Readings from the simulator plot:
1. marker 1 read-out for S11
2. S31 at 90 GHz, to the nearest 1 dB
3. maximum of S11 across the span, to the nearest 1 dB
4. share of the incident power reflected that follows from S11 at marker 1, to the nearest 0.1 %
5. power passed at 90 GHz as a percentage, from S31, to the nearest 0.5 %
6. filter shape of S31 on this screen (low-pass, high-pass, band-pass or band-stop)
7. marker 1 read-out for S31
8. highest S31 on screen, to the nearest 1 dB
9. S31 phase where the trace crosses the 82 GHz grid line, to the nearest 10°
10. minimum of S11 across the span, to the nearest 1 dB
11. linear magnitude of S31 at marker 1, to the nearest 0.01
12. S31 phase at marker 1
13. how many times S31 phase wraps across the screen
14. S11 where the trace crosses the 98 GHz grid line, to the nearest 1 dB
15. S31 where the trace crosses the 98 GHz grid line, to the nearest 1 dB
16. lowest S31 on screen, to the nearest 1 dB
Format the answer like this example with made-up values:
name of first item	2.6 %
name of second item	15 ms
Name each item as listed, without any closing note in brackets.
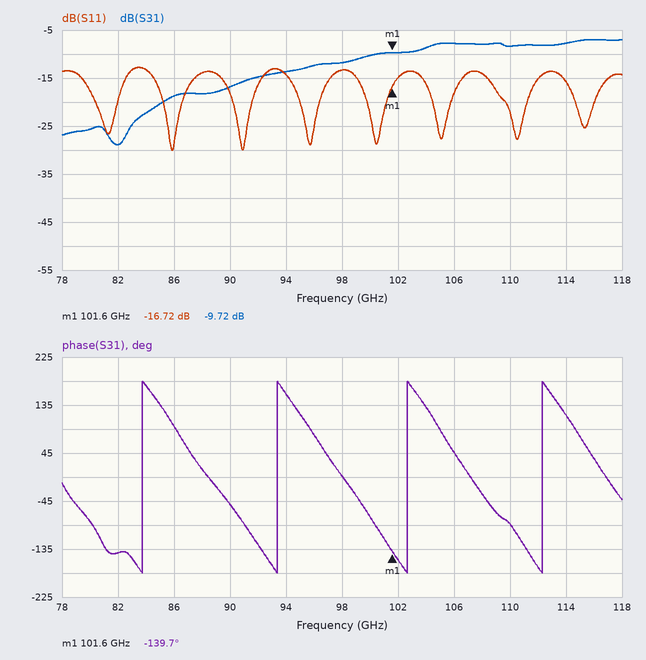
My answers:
marker 1 read-out for S11	-16.72 dB
S31 at 90 GHz, to the nearest 1 dB	-17 dB
maximum of S11 across the span, to the nearest 1 dB	-13 dB
share of the incident power reflected that follows from S11 at marker 1, to the nearest 0.1 %	2.1 %
power passed at 90 GHz as a percentage, from S31, to the nearest 0.5 %	2.0 %
filter shape of S31 on this screen	high-pass
marker 1 read-out for S31	-9.72 dB
highest S31 on screen, to the nearest 1 dB	-7 dB
S31 phase where the trace crosses the 82 GHz grid line, to the nearest 10°	-140°
minimum of S11 across the span, to the nearest 1 dB	-30 dB
linear magnitude of S31 at marker 1, to the nearest 0.01	0.33
S31 phase at marker 1	-139.7°
how many times S31 phase wraps across the screen	4
S11 where the trace crosses the 98 GHz grid line, to the nearest 1 dB	-13 dB
S31 where the trace crosses the 98 GHz grid line, to the nearest 1 dB	-12 dB
lowest S31 on screen, to the nearest 1 dB	-29 dB
